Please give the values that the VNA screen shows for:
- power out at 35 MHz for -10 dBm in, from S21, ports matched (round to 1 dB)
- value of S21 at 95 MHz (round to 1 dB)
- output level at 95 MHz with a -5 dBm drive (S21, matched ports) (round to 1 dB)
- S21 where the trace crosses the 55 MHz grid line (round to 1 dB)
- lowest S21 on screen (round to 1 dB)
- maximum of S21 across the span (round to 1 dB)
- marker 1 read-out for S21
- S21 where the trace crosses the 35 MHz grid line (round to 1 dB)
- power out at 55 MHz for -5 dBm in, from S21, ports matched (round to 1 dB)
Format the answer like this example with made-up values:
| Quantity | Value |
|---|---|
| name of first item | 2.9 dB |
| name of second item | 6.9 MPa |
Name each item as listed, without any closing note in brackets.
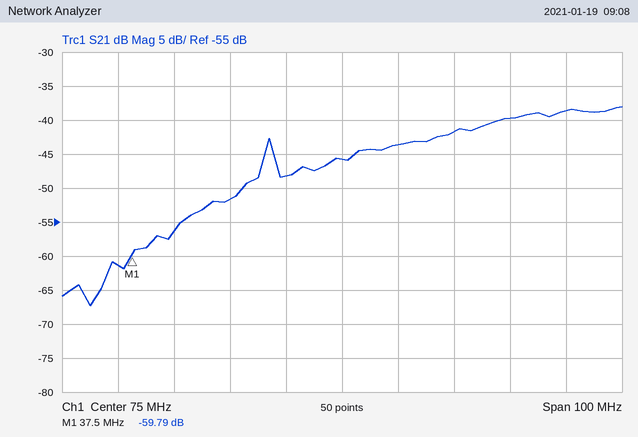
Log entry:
| Quantity | Value |
|---|---|
| power out at 35 MHz for -10 dBm in, from S21, ports matched | -71 dBm |
| value of S21 at 95 MHz | -42 dB |
| output level at 95 MHz with a -5 dBm drive (S21, matched ports) | -47 dBm |
| S21 where the trace crosses the 55 MHz grid line | -52 dB |
| lowest S21 on screen | -67 dB |
| maximum of S21 across the span | -38 dB |
| marker 1 read-out for S21 | -59.79 dB |
| S21 where the trace crosses the 35 MHz grid line | -61 dB |
| power out at 55 MHz for -5 dBm in, from S21, ports matched | -57 dBm |
